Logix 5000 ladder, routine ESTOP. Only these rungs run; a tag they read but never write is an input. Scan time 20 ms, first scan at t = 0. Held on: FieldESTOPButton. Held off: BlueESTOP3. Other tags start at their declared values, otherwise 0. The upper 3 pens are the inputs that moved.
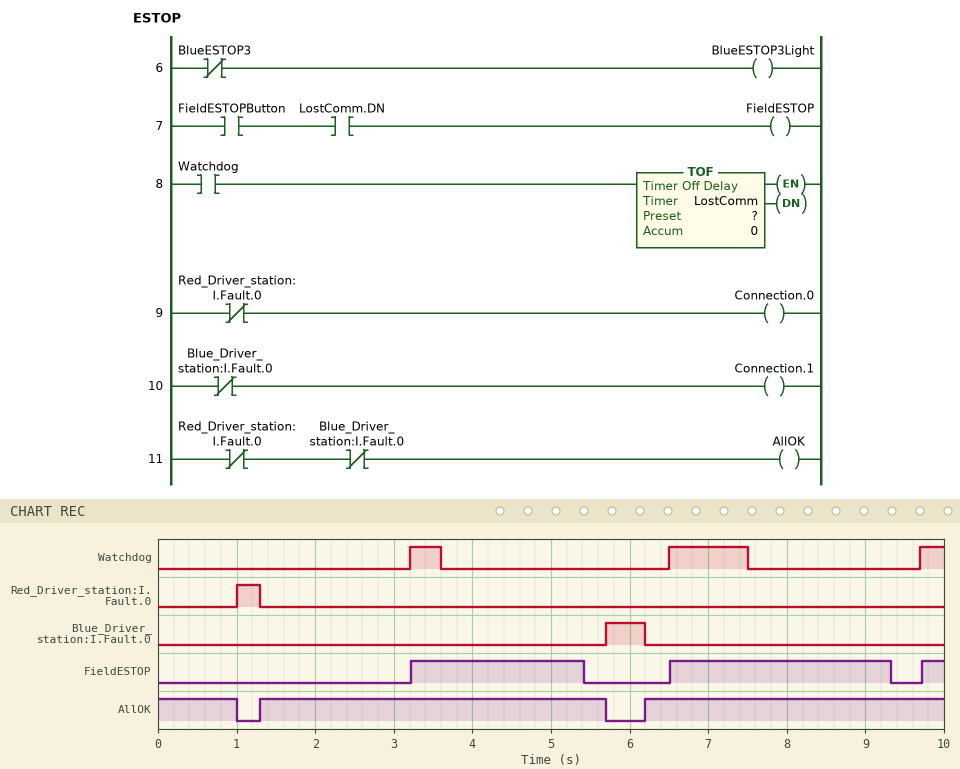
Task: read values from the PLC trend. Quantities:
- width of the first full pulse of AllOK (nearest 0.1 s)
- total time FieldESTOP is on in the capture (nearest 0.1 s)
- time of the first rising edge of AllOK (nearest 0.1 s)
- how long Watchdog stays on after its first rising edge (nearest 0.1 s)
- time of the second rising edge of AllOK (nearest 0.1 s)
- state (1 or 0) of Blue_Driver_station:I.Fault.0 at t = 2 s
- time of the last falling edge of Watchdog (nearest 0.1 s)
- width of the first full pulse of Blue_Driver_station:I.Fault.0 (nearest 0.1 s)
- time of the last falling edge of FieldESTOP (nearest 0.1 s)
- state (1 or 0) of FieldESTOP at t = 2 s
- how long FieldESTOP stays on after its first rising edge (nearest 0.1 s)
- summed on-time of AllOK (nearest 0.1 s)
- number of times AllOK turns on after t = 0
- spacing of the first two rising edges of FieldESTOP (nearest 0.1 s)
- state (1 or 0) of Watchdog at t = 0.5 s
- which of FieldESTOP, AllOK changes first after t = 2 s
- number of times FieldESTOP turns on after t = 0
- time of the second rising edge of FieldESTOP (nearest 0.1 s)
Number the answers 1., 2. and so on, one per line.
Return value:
1. 4.4 s
2. 5.3 s
3. 1.3 s
4. 0.4 s
5. 6.2 s
6. 0
7. 7.5 s
8. 0.5 s
9. 9.3 s
10. 0
11. 2.2 s
12. 9.2 s
13. 2
14. 3.3 s
15. 0
16. FieldESTOP
17. 3
18. 6.5 s
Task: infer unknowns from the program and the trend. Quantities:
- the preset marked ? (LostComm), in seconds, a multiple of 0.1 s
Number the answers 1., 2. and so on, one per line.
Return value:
1. 1.8 s
